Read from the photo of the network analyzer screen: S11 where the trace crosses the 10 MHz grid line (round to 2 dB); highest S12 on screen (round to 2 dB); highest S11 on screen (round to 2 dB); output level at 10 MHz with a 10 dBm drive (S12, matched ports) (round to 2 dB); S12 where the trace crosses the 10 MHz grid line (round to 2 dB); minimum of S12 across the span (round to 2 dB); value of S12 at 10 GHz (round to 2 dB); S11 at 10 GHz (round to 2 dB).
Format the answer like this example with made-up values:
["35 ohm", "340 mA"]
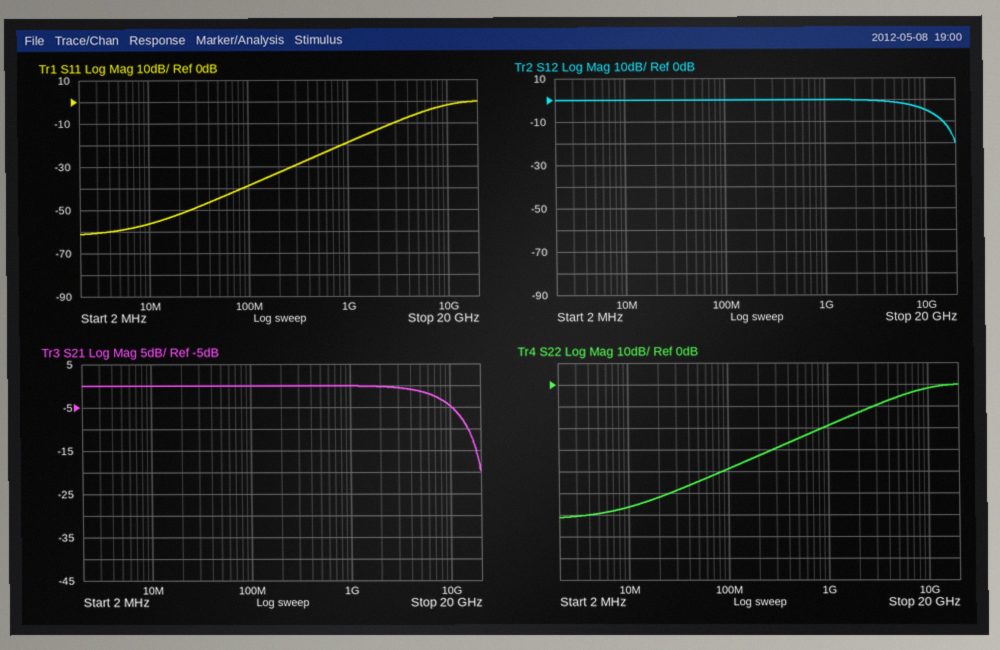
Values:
["-56 dB", "0 dB", "0 dB", "10 dBm", "0 dB", "-20 dB", "-4 dB", "-2 dB"]
